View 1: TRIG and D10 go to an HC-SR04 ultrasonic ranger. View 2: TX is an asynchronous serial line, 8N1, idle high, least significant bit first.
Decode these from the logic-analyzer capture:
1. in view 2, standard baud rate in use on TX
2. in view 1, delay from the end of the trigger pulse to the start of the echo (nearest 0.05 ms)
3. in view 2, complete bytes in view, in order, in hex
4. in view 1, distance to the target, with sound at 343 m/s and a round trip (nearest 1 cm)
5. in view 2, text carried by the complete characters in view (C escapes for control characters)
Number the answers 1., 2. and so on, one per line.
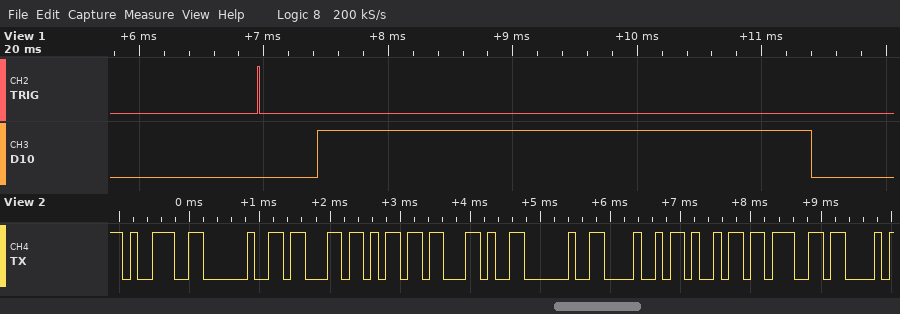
1. 9600 baud
2. 0.45 ms
3. 0x39 0x20 0x63 0x6D 0x2C 0x20 0x48 0x69 0x67
4. 68 cm
5. "9 cm, Hig"
